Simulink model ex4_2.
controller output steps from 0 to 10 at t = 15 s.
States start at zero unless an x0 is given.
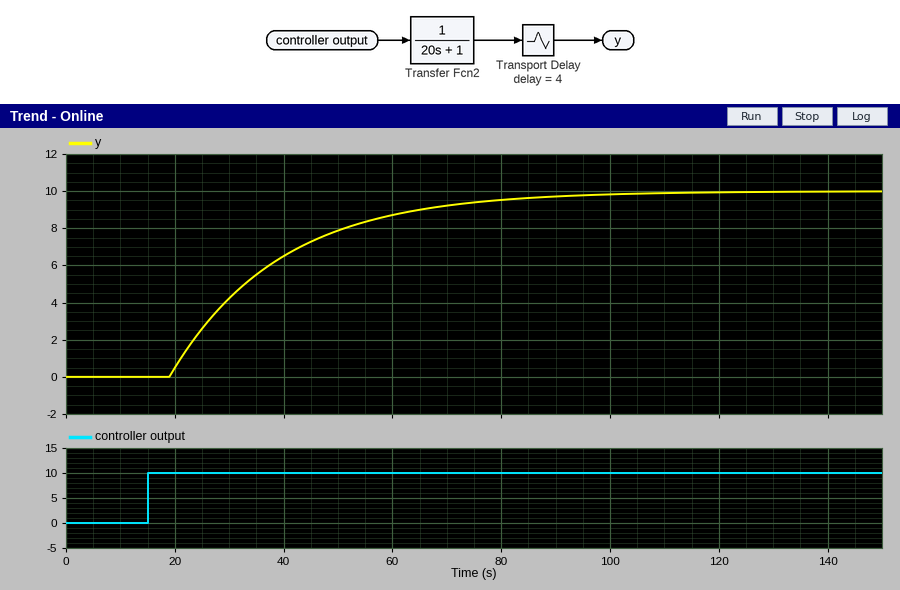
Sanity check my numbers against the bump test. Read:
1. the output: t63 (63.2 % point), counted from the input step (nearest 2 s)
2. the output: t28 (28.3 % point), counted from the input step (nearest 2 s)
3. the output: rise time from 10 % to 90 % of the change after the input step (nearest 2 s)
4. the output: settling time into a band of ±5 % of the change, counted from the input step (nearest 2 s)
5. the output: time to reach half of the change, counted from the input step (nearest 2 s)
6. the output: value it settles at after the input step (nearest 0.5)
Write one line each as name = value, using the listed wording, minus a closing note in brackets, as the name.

the output: t63 (63.2 % point), counted from the input step = 24 s
the output: t28 (28.3 % point), counted from the input step = 10 s
the output: rise time from 10 % to 90 % of the change after the input step = 44 s
the output: settling time into a band of ±5 % of the change, counted from the input step = 64 s
the output: time to reach half of the change, counted from the input step = 18 s
the output: value it settles at after the input step = 10.0
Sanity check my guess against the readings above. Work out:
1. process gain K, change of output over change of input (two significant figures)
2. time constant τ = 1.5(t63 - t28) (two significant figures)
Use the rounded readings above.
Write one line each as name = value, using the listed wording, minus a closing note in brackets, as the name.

process gain K, change of output over change of input = 1.0
time constant τ = 1.5(t63 - t28) = 21 s
